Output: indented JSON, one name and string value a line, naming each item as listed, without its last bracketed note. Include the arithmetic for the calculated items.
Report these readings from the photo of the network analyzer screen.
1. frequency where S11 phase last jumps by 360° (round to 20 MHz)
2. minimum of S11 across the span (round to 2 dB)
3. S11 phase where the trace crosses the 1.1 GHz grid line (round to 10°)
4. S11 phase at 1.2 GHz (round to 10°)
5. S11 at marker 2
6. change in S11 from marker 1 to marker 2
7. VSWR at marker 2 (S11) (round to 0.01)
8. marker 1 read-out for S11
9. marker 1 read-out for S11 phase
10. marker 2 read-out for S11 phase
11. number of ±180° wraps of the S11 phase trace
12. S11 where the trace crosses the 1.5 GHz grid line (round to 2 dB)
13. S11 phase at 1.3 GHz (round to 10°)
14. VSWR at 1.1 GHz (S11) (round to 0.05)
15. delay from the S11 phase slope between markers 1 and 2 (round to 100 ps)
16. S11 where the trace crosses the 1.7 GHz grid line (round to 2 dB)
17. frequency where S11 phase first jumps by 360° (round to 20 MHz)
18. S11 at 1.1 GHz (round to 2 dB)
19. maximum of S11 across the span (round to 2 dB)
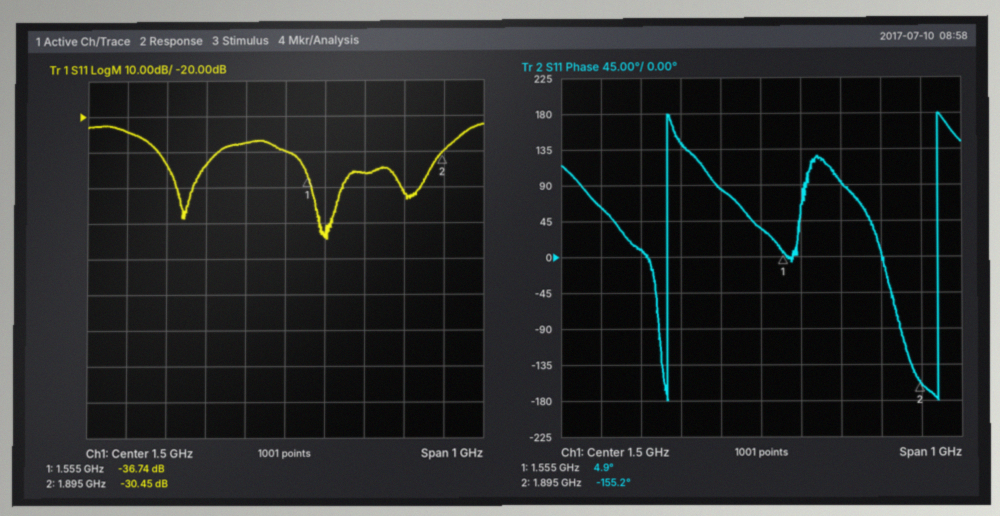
{
  "frequency where S11 phase last jumps by 360°": "1.94 GHz",
  "minimum of S11 across the span": "-54 dB",
  "S11 phase where the trace crosses the 1.1 GHz grid line": "60°",
  "S11 phase at 1.2 GHz": "10°",
  "S11 at marker 2": "-30.45 dB",
  "change in S11 from marker 1 to marker 2": "-30.45 − (-36.74) = 6.29 dB",
  "VSWR at marker 2 (S11)": "(1 + 0.0300)/(1 − 0.0300) ≈ 1.06",
  "marker 1 read-out for S11": "-36.74 dB",
  "marker 1 read-out for S11 phase": "4.9°",
  "marker 2 read-out for S11 phase": "-155.2°",
  "number of ±180° wraps of the S11 phase trace": "2",
  "S11 where the trace crosses the 1.5 GHz grid line": "-30 dB",
  "S11 phase at 1.3 GHz": "140°",
  "VSWR at 1.1 GHz (S11)": "|Γ| = 10^(-24/20) = 0.0631; VSWR = (1 + 0.0631)/(1 − 0.0631) ≈ 1.13, so 1.15 to the nearest 0.05",
  "delay from the S11 phase slope between markers 1 and 2": "−(-155.2° − (4.9°))/(360° × 340 MHz) ≈ 1.3 ns",
  "S11 where the trace crosses the 1.7 GHz grid line": "-36 dB",
  "frequency where S11 phase first jumps by 360°": "1.26 GHz",
  "S11 at 1.1 GHz": "-24 dB",
  "maximum of S11 across the span": "-22 dB"
}
